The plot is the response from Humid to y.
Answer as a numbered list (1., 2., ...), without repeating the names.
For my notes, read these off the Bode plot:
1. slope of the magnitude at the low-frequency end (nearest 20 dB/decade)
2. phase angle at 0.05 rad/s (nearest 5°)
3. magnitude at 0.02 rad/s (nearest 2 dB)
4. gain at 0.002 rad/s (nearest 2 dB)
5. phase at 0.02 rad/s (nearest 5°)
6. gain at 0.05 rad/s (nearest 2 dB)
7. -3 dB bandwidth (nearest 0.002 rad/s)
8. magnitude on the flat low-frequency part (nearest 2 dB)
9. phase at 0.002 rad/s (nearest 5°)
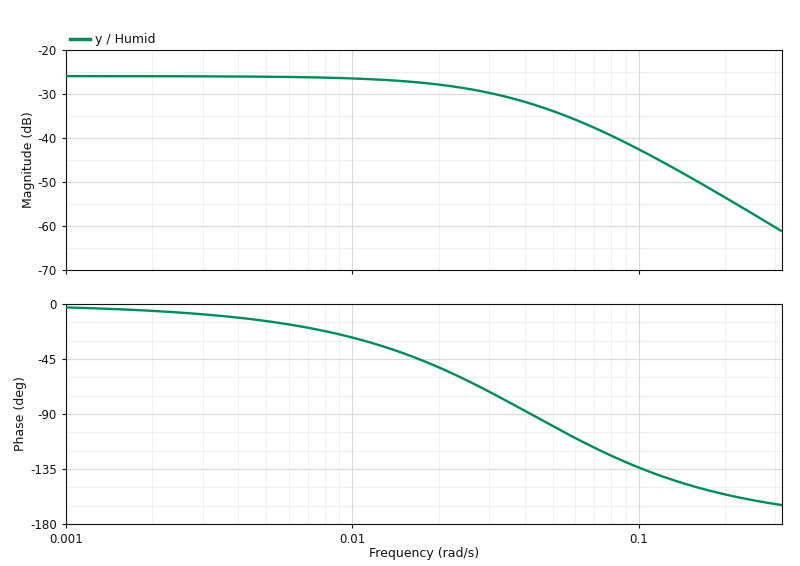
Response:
1. 0 dB/decade
2. -100°
3. -28 dB
4. -26 dB
5. -50°
6. -34 dB
7. 0.026 rad/s
8. -26 dB
9. -5°
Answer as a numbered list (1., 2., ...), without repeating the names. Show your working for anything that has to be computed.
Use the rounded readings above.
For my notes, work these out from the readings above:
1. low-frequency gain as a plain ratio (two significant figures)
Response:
1. 10^(-26 / 20) = 0.050
